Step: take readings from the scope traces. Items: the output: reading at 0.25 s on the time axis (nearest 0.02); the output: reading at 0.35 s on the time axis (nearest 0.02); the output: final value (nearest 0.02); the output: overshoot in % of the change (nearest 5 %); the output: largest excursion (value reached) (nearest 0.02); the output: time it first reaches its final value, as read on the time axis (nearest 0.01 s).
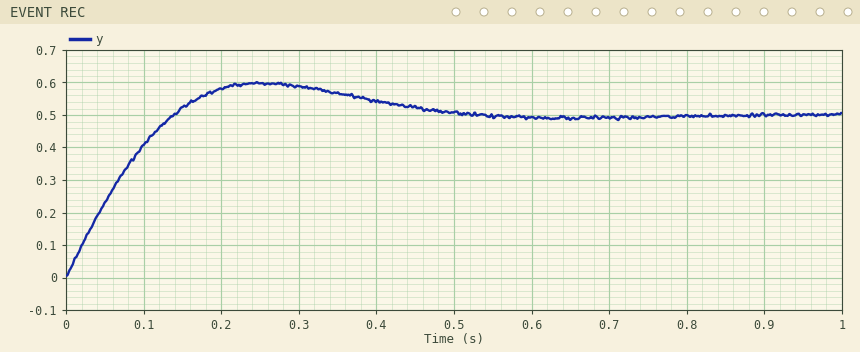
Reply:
0.60
0.56
0.50
20 %
0.60
0.14 s
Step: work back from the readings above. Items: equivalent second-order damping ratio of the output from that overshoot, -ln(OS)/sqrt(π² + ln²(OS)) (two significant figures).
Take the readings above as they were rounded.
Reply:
0.46
